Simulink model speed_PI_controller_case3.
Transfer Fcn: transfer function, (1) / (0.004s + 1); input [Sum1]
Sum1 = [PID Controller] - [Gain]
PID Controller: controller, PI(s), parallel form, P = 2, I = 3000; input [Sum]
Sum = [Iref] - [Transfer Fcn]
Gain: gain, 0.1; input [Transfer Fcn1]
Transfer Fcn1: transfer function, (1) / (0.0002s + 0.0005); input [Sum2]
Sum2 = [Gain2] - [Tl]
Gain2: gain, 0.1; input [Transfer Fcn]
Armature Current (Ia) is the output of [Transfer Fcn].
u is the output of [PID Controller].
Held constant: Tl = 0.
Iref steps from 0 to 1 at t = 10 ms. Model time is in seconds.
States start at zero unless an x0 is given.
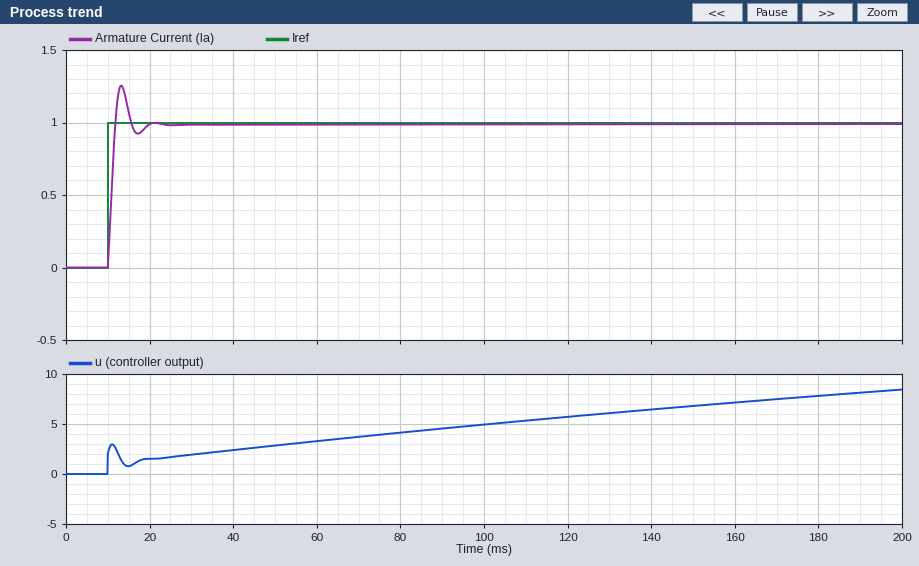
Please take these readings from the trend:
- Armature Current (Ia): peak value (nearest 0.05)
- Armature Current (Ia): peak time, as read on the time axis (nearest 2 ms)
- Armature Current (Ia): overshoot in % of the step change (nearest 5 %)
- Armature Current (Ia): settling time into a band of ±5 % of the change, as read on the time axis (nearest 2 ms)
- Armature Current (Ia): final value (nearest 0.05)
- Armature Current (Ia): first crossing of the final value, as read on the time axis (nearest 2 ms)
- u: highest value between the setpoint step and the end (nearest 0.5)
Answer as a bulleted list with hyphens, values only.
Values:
- 1.25
- 14 ms
- 25 %
- 18 ms
- 1.00
- 12 ms
- 8.5
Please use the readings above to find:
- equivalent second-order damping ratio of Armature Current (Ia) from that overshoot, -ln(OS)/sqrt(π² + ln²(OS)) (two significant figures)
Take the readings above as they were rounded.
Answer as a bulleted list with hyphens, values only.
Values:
- 0.40
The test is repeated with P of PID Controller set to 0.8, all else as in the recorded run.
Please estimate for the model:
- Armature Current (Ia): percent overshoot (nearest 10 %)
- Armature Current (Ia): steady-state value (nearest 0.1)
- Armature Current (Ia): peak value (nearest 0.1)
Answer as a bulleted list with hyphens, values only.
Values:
- 40 %
- 1.0
- 1.4
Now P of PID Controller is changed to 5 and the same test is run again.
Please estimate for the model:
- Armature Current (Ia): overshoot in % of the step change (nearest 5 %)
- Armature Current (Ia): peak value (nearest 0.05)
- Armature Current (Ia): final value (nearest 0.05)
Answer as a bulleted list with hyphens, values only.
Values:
- 10 %
- 1.10
- 1.00
